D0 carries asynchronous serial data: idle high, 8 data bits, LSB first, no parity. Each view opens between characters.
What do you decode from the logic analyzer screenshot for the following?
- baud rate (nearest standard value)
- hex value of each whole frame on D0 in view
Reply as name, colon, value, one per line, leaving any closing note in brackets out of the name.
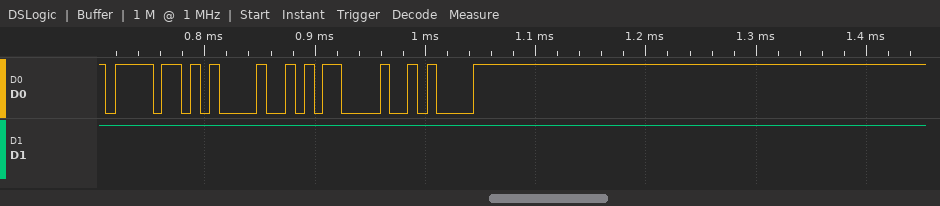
baud rate: 115200 baud
hex value of each whole frame on D0 in view: 6F, 21, 0D, 0A
